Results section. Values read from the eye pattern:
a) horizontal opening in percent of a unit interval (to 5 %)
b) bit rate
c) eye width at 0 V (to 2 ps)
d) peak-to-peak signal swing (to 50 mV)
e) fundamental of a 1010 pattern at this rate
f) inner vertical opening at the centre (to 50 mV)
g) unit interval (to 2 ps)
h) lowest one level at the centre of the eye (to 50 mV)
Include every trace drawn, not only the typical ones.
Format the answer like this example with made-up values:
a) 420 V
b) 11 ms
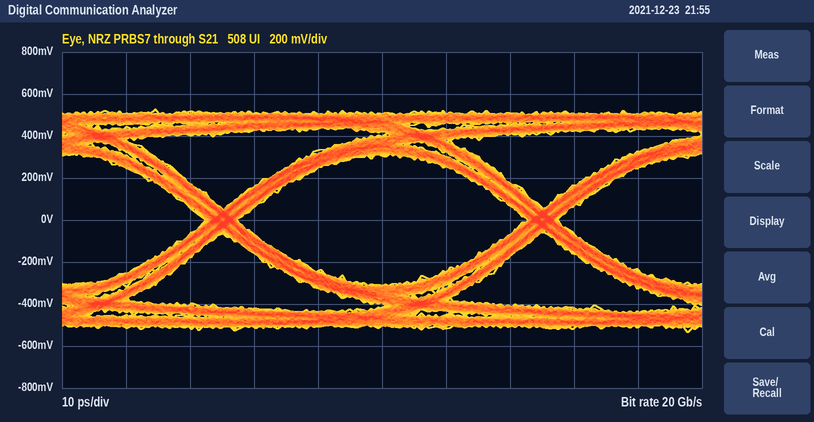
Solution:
a) 90 %
b) 20 Gb/s
c) 46 ps
d) 1.05 V
e) 10 GHz
f) 600 mV
g) 50 ps
h) 300 mV
